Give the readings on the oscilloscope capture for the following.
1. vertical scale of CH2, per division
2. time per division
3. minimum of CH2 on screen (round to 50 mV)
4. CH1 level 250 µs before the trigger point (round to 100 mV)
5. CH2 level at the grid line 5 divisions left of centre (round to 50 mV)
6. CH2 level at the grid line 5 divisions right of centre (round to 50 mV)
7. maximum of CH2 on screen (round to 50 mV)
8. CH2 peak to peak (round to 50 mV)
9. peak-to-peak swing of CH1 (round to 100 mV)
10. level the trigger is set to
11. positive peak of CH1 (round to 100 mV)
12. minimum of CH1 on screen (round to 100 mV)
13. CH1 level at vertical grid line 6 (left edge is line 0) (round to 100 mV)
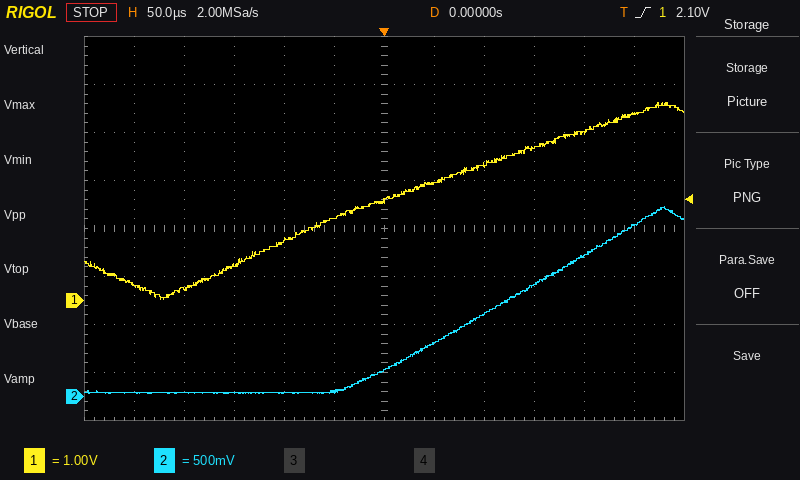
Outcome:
500 mV
50 µs
50 mV
300 mV
50 mV
1.80 V
2.00 V
1.95 V
4.1 V
2.10 V
4.1 V
0.0 V
2.1 V
